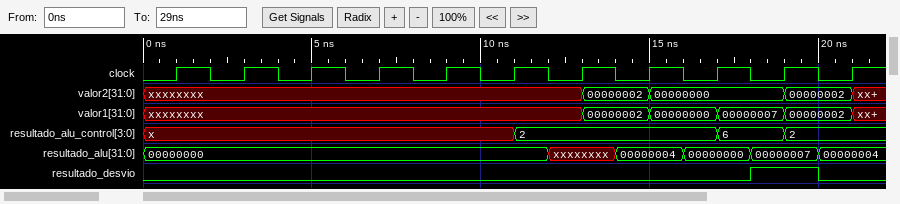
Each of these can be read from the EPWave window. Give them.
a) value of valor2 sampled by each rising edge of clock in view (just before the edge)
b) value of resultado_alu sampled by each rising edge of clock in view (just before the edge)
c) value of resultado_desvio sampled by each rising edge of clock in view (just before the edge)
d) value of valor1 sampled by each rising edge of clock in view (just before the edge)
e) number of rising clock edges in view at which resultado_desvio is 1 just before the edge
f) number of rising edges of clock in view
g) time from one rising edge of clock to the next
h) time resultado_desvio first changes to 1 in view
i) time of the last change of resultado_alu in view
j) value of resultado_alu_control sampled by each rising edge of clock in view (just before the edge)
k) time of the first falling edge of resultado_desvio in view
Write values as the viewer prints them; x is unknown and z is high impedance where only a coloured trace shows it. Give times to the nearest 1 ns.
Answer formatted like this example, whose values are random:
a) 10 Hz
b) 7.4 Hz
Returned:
a) xxxxxxxx, xxxxxxxx, xxxxxxxx, xxxxxxxx, xxxxxxxx, xxxxxxxx, xxxxxxxx, 00000002, 00000000, 00000000, 00000002
b) 00000000, 00000000, 00000000, 00000000, 00000000, 00000000, xxxxxxxx, 00000004, 00000000, 00000007, 00000004
c) 0 0 0 0 0 0 0 0 0 1 0
d) xxxxxxxx, xxxxxxxx, xxxxxxxx, xxxxxxxx, xxxxxxxx, xxxxxxxx, xxxxxxxx, 00000002, 00000000, 00000007, 00000002
e) 1
f) 11
g) 2 ns
h) 18 ns
i) 20 ns
j) x, x, x, x, x, x, 2, 2, 2, 6, 2
k) 20 ns
